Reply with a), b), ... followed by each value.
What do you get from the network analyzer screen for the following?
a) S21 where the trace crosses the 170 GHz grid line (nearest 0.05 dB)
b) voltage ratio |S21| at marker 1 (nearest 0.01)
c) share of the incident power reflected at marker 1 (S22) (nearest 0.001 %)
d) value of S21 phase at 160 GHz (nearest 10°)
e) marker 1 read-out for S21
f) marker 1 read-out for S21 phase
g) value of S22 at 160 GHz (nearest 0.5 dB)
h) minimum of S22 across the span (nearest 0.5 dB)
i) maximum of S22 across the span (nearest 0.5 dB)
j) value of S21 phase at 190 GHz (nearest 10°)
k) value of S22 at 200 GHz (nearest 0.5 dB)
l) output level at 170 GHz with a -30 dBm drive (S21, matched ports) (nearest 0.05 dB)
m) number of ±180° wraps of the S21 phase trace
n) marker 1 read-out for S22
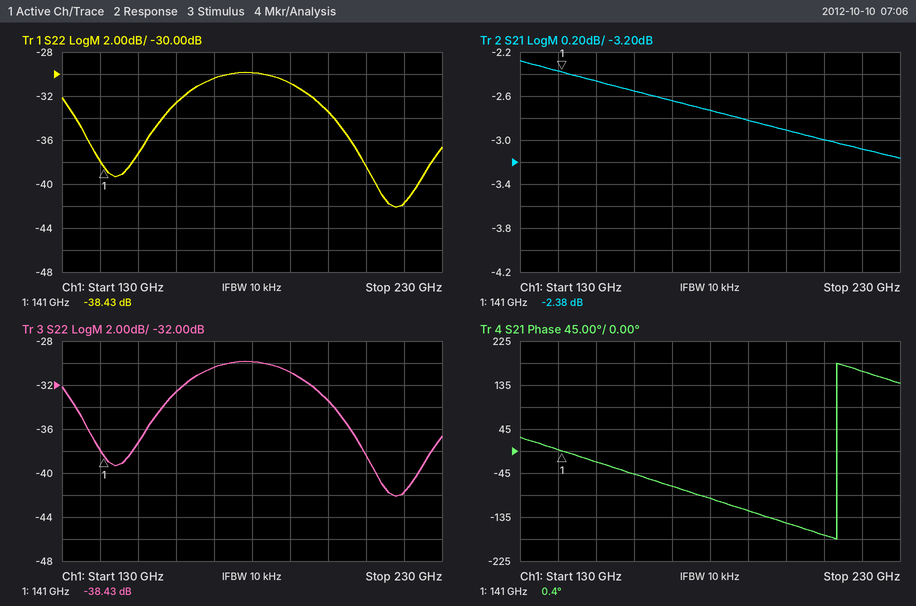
a) -2.65 dB
b) 0.76
c) 0.014 %
d) -50°
e) -2.38 dB
f) 0.4°
g) -32.5 dB
h) -42.0 dB
i) -30.0 dB
j) -120°
k) -33.5 dB
l) -32.65 dBm
m) 1
n) -38.43 dB
